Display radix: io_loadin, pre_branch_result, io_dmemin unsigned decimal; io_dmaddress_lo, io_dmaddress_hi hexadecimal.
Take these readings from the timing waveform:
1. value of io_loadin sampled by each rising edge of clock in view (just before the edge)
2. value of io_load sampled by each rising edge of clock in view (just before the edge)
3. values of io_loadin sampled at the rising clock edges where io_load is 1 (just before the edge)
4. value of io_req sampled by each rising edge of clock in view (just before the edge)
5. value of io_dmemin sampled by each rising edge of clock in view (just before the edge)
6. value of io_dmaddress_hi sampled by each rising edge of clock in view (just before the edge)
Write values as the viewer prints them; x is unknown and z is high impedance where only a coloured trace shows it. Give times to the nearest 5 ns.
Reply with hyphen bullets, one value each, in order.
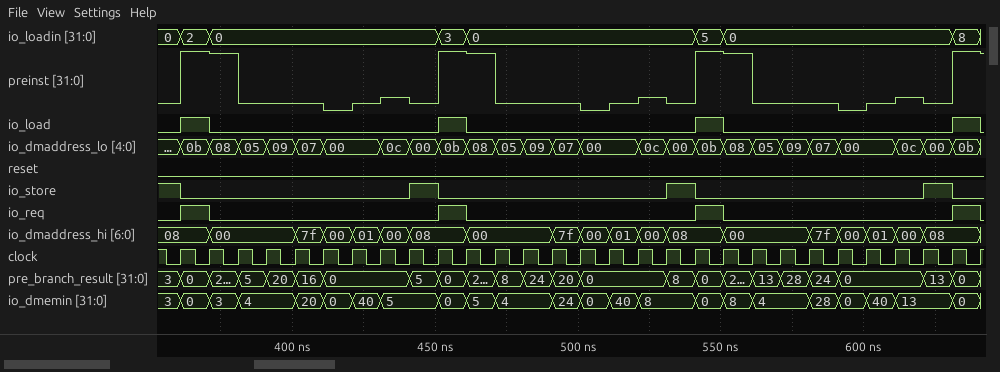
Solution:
- 0, 2, 0, 0, 0, 0, 0, 0, 0, 0, 3, 0, 0, 0, 0, 0, 0, 0, 0, 5, 0, 0, 0, 0, 0, 0, 0, 0, 8
- 0 1 0 0 0 0 0 0 0 0 1 0 0 0 0 0 0 0 0 1 0 0 0 0 0 0 0 0 1
- 2, 3, 5, 8
- 0 1 0 0 0 0 0 0 0 0 1 0 0 0 0 0 0 0 0 1 0 0 0 0 0 0 0 0 1
- 3, 0, 3, 4, 4, 20, 0, 40, 5, 5, 0, 5, 4, 4, 24, 0, 40, 8, 8, 0, 8, 4, 4, 28, 0, 40, 13, 13, 0
- 08, 08, 00, 00, 00, 7f, 00, 01, 00, 08, 08, 00, 00, 00, 7f, 00, 01, 00, 08, 08, 00, 00, 00, 7f, 00, 01, 00, 08, 08
